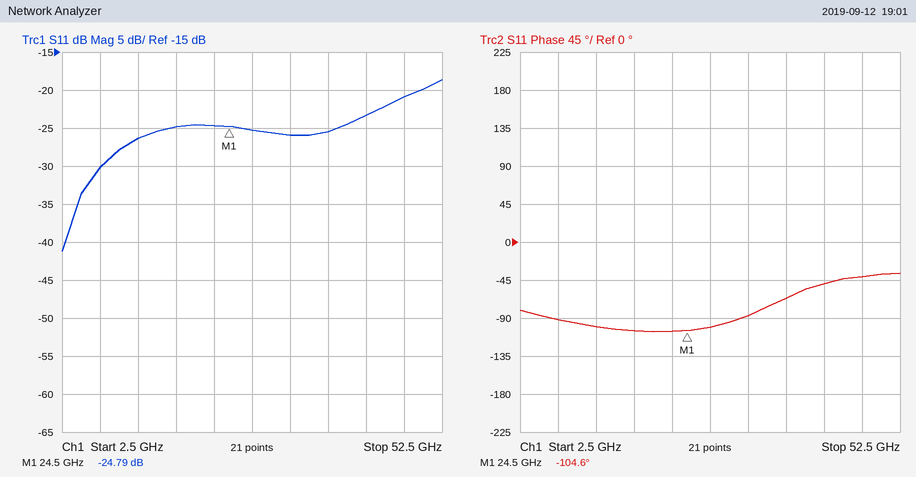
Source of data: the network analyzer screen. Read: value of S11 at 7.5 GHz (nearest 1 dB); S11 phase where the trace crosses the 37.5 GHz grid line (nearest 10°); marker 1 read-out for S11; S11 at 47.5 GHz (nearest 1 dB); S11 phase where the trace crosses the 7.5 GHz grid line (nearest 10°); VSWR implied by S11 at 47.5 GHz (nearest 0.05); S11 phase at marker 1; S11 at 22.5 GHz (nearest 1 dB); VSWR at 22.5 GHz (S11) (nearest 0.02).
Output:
-30 dB
-70°
-24.79 dB
-21 dB
-90°
1.20
-104.6°
-25 dB
1.12
